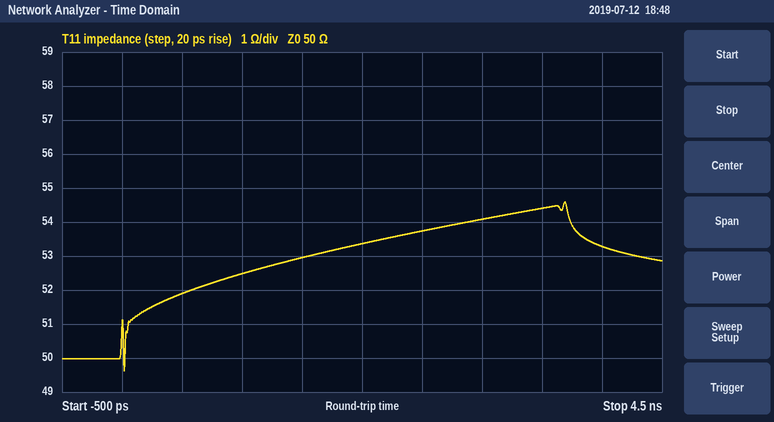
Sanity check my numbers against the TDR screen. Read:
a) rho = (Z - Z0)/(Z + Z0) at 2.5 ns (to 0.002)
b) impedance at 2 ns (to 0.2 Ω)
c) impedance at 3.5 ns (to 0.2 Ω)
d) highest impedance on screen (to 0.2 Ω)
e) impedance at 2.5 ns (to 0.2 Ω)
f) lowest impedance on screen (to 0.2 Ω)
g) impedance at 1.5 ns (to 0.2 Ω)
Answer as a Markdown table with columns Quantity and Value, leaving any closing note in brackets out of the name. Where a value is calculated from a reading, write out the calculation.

| Quantity | Value |
|---|---|
| rho = (Z - Z0)/(Z + Z0) at 2.5 ns | (53.8 − 50)/(53.8 + 50) ≈ +0.0366, so +0.036 to the nearest 0.002 |
| impedance at 2 ns | 53.4 Ω |
| impedance at 3.5 ns | 54.4 Ω |
| highest impedance on screen | 54.6 Ω |
| impedance at 2.5 ns | 53.8 Ω |
| lowest impedance on screen | 49.6 Ω |
| impedance at 1.5 ns | 53.0 Ω |
